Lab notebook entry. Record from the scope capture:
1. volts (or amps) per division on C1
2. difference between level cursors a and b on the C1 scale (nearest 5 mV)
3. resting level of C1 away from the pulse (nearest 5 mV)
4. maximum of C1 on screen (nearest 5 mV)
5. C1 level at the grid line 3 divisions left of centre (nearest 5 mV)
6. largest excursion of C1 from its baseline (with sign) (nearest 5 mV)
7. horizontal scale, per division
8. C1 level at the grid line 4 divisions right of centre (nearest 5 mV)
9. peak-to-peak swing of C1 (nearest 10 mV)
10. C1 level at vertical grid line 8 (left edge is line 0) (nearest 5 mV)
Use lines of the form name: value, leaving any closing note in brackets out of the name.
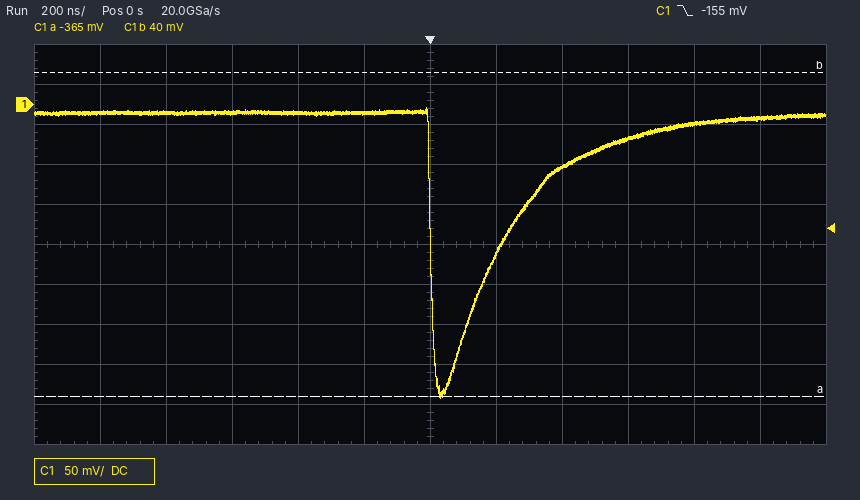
volts (or amps) per division on C1: 50 mV
difference between level cursors a and b on the C1 scale: 405 mV
resting level of C1 away from the pulse: -10 mV
maximum of C1 on screen: -5 mV
C1 level at the grid line 3 divisions left of centre: -10 mV
largest excursion of C1 from its baseline (with sign): -355 mV
horizontal scale, per division: 200 ns
C1 level at the grid line 4 divisions right of centre: -25 mV
peak-to-peak swing of C1: 360 mV
C1 level at vertical grid line 8 (left edge is line 0): -80 mV
